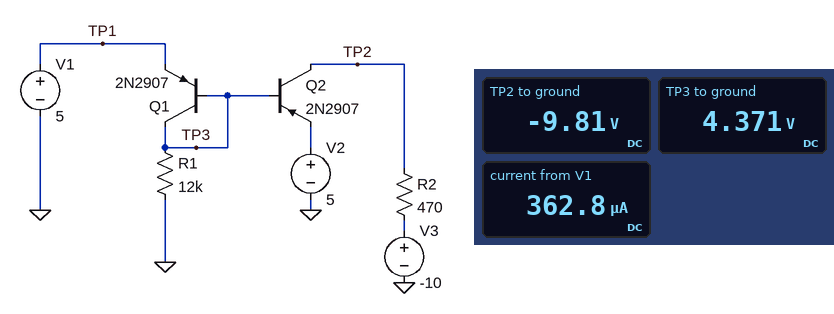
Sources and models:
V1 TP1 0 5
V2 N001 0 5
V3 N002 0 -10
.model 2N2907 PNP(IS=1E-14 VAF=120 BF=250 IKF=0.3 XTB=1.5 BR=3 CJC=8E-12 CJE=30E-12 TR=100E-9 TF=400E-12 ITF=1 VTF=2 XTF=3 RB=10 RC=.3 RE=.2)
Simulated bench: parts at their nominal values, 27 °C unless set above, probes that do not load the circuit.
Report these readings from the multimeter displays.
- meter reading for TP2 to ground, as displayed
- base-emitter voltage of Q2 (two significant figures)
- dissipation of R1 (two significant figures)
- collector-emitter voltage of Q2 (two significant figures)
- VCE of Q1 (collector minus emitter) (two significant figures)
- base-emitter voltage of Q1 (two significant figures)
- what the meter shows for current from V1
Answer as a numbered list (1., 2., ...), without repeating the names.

1. -9.81 V
2. -630 mV
3. 1.6 mW
4. -15 V
5. -630 mV
6. -630 mV
7. 362.8 µA
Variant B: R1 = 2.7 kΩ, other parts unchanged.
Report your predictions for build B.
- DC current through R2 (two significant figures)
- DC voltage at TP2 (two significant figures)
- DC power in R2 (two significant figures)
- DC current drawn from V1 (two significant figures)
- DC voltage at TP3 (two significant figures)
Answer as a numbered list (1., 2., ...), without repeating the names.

1. 1.8 mA
2. -9.2 V
3. 1.5 mW
4. 1.6 mA
5. 4.3 V
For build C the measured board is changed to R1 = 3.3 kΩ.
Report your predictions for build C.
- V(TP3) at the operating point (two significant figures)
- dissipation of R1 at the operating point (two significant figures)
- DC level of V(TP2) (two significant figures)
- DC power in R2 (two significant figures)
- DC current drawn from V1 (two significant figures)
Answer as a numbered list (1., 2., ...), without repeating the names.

1. 4.3 V
2. 5.7 mW
3. -9.3 V
4. 990 µW
5. 1.3 mA
